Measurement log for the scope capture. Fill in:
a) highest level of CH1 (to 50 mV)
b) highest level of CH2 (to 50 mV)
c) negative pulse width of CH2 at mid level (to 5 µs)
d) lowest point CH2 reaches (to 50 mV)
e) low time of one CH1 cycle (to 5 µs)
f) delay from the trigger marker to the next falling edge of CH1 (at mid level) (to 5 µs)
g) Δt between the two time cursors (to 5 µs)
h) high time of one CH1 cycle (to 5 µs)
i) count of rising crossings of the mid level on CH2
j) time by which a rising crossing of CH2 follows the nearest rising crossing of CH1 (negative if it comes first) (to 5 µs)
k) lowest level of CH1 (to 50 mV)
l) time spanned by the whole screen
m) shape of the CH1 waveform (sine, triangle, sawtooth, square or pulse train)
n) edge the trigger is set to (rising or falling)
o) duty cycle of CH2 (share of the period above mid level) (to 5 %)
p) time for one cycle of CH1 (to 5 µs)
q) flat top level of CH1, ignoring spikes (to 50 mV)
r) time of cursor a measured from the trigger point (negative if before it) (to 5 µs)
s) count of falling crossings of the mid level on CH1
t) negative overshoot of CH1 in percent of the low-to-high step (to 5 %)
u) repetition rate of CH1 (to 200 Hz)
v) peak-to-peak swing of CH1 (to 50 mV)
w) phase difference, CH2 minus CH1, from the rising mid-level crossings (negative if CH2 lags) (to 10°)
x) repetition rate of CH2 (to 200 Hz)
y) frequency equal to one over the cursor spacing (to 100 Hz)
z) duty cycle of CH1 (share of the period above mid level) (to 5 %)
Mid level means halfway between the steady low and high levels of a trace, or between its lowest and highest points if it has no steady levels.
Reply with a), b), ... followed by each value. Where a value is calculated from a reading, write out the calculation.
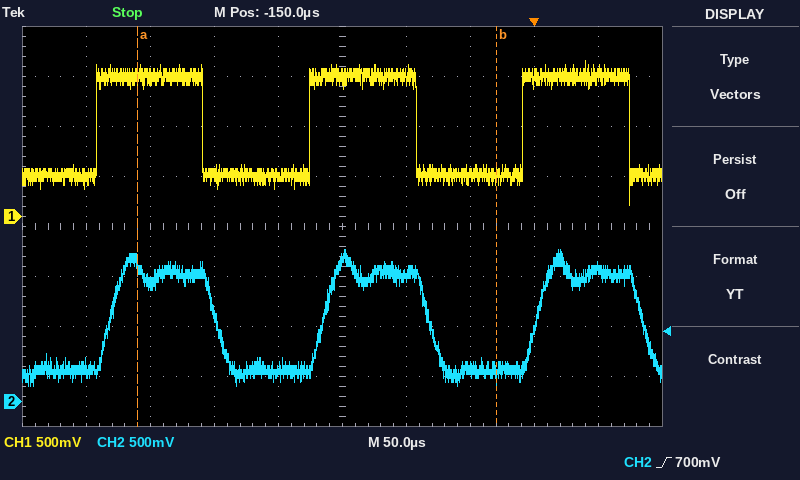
a) 1.55 V
b) 1.50 V
c) 85 µs
d) 150 mV
e) 85 µs
f) 75 µs
g) 280 µs
h) 85 µs
i) 3
j) +10 µs
k) 100 mV
l) 500 µs
m) square
n) rising
o) 50 %
p) 165 µs
q) 1.40 V
r) -310 µs
s) 3
t) 30 %
u) 1 / 165 µs ≈ 6.06 kHz, so 6.0 kHz to the nearest 200 Hz
v) 1.55 V − (100 mV) = 1.45 V
w) −360° × (+10 µs) / 165 µs ≈ -21.8°, so -20° to the nearest 10°
x) 1 / 165 µs ≈ 6.06 kHz, so 6.0 kHz to the nearest 200 Hz
y) 1 / 280 µs ≈ 3.6 kHz
z) 85 µs / 165 µs ≈ 51.5 %, so 50 % to the nearest 5 %
